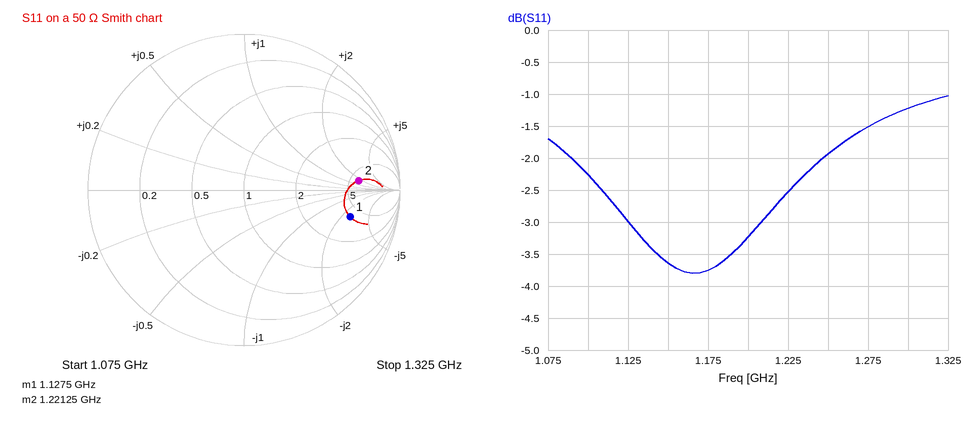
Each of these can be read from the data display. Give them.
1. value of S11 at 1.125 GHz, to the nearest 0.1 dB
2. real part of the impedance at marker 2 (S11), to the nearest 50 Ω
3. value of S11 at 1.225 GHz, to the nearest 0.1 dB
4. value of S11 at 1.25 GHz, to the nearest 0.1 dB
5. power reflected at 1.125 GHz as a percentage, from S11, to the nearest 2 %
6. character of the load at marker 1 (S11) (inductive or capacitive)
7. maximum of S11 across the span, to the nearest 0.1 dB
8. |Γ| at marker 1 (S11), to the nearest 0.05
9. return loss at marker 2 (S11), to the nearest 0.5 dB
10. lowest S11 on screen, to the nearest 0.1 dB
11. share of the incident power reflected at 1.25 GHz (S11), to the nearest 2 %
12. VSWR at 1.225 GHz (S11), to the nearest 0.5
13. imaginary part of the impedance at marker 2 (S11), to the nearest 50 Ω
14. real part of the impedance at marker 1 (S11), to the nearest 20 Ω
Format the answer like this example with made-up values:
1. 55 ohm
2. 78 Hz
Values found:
1. -3.0 dB
2. 300 Ω
3. -2.5 dB
4. -1.9 dB
5. 50 %
6. capacitive
7. -1.0 dB
8. 0.70
9. 2.5 dB
10. -3.8 dB
11. 64 %
12. 7.0
13. +100 Ω
14. 200 Ω
